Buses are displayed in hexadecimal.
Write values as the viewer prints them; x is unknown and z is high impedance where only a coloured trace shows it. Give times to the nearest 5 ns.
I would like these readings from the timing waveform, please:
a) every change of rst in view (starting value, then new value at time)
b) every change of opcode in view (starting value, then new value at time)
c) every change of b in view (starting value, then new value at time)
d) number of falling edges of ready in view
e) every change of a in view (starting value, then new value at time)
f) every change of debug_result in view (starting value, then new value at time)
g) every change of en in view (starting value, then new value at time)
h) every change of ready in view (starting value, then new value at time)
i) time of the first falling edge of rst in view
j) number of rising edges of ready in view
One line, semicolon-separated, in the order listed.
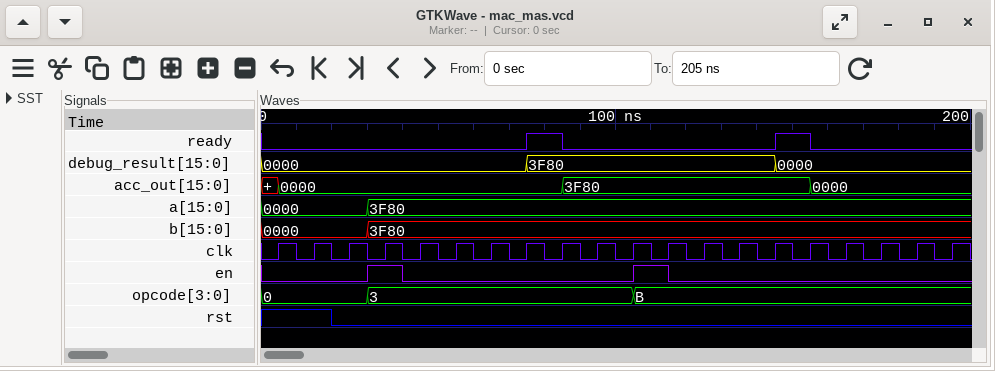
1, 0 at 20 ns; 0, 3 at 30 ns, B at 105 ns; 0000, 3F80 at 30 ns; 2; 0000, 3F80 at 30 ns; 0000, 3F80 at 75 ns, 0000 at 145 ns; 0, 1 at 30 ns, 0 at 40 ns, 1 at 105 ns, 0 at 115 ns; 0, 1 at 75 ns, 0 at 85 ns, 1 at 145 ns, 0 at 155 ns; 20 ns; 2
